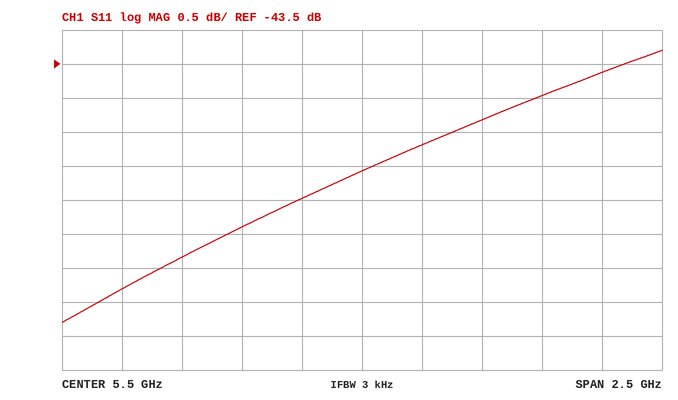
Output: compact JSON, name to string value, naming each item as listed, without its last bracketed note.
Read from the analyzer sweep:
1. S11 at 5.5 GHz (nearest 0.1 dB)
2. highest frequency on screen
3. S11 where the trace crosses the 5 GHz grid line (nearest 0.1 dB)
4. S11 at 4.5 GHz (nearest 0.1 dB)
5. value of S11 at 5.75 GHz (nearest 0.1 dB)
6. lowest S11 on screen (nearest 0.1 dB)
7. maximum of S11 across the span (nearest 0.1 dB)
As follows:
{"S11 at 5.5 GHz": "-45.1 dB", "highest frequency on screen": "6.75 GHz", "S11 where the trace crosses the 5 GHz grid line": "-45.9 dB", "S11 at 4.5 GHz": "-46.8 dB", "value of S11 at 5.75 GHz": "-44.7 dB", "lowest S11 on screen": "-47.3 dB", "maximum of S11 across the span": "-43.3 dB"}
